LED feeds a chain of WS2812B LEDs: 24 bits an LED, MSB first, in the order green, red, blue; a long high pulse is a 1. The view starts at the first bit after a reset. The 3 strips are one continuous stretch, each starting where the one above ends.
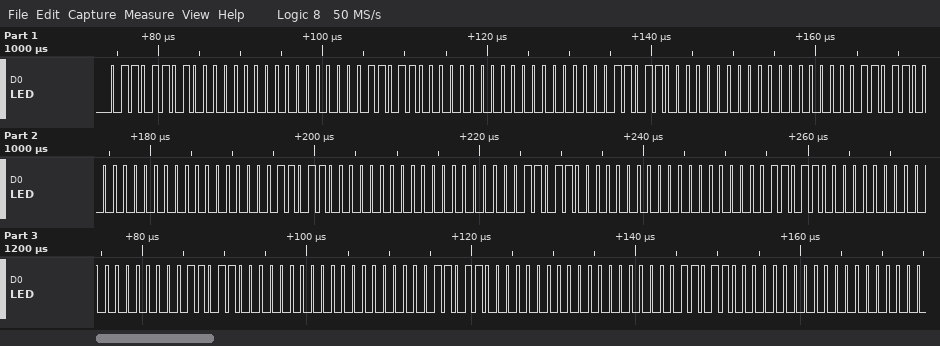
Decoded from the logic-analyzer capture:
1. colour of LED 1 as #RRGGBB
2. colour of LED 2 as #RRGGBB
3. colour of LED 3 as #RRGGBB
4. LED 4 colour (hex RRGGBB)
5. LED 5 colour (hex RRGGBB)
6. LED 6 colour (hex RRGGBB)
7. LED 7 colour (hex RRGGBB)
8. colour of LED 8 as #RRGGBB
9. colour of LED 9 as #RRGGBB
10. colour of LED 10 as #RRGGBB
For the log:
#006D00
#006C00
#006C00
#006C00
#006C00
#006C00
#006C00
#006C00
#006C00
#006C00
